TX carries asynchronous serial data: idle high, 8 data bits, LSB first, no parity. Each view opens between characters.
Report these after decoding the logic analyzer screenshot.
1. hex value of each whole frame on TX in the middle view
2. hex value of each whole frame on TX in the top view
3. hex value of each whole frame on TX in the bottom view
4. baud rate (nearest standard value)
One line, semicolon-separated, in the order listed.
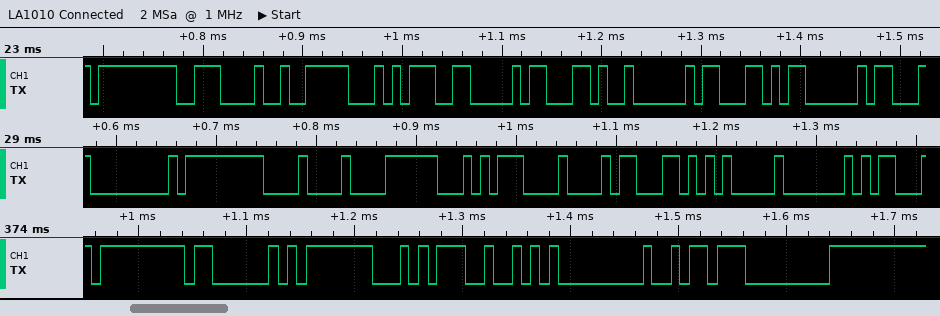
00, FF, 08, F8, D4, 08, 63, 05, 40; FF, 0E, F2, D4, 06, 63, 02, 63, 03; FF, 03, FD, D4, 52, 00, DA, 00; 115200 baud
